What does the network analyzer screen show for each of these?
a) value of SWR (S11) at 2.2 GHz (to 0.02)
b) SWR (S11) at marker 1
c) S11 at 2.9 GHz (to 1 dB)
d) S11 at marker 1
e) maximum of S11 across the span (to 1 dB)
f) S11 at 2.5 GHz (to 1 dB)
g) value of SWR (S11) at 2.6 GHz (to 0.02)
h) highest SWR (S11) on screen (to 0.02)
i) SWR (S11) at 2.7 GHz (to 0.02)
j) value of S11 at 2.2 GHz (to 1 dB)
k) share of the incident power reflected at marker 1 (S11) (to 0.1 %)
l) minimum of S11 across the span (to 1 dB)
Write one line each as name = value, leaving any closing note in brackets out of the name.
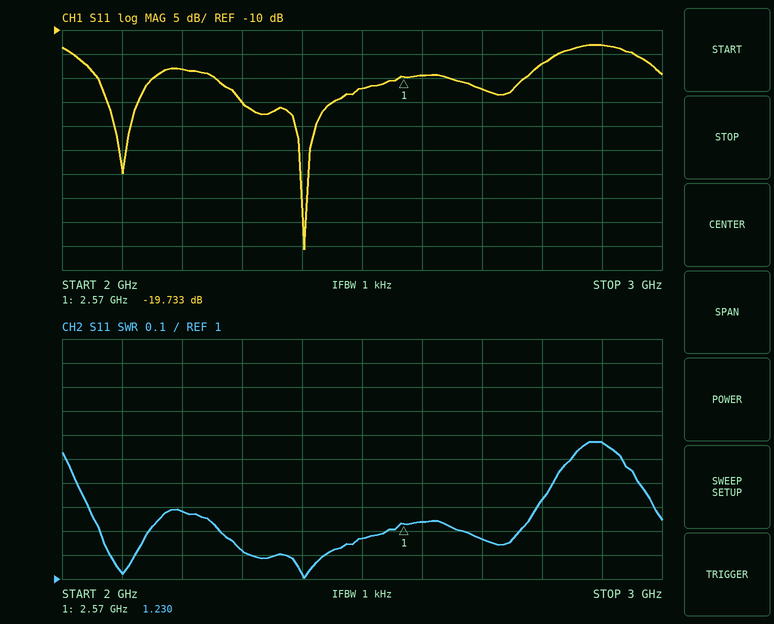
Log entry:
value of SWR (S11) at 2.2 GHz = 1.28
SWR (S11) at marker 1 = 1.230
S11 at 2.9 GHz = -13 dB
S11 at marker 1 = -19.733 dB
maximum of S11 across the span = -13 dB
S11 at 2.5 GHz = -22 dB
value of SWR (S11) at 2.6 GHz = 1.24
highest SWR (S11) on screen = 1.58
SWR (S11) at 2.7 GHz = 1.16
value of S11 at 2.2 GHz = -18 dB
share of the incident power reflected at marker 1 (S11) = 1.1 %
minimum of S11 across the span = -56 dB
